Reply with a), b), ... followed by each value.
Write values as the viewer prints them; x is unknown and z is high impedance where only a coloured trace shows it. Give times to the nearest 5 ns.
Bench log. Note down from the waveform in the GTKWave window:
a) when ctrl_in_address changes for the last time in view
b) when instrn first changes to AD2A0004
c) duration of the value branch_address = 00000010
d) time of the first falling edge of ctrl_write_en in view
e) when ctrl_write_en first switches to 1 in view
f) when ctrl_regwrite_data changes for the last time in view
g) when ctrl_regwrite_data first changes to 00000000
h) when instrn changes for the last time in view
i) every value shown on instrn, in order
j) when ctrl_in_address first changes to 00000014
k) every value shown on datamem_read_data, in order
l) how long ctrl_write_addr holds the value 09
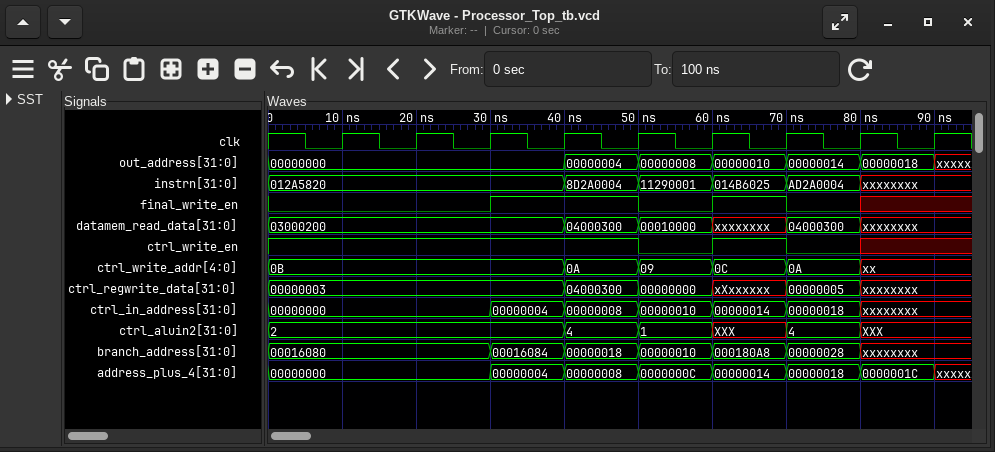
a) 80 ns
b) 70 ns
c) 10 ns
d) 50 ns
e) 60 ns
f) 80 ns
g) 50 ns
h) 80 ns
i) 012A5820, 8D2A0004, 11290001, 014B6025, AD2A0004, xxxxxxxx
j) 60 ns
k) 03000200, 04000300, 00010000, xxxxxxxx, 04000300, xxxxxxxx
l) 10 ns
